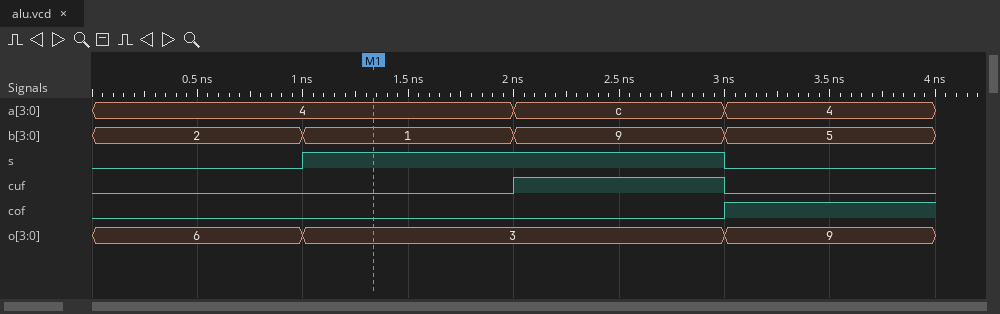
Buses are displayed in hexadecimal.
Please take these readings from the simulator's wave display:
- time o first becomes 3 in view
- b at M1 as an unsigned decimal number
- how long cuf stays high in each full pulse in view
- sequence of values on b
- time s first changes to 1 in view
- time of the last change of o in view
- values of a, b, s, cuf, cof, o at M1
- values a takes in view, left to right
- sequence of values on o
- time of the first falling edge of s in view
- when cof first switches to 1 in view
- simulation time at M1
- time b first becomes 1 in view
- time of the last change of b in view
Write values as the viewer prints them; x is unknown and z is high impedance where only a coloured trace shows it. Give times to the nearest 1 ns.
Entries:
1 ns
1
1 ns
2, 1, 9, 5
1 ns
3 ns
a=4, b=1, s=1, cuf=0, cof=0, o=3
4, c, 4
6, 3, 9
3 ns
3 ns
1 ns
1 ns
3 ns
